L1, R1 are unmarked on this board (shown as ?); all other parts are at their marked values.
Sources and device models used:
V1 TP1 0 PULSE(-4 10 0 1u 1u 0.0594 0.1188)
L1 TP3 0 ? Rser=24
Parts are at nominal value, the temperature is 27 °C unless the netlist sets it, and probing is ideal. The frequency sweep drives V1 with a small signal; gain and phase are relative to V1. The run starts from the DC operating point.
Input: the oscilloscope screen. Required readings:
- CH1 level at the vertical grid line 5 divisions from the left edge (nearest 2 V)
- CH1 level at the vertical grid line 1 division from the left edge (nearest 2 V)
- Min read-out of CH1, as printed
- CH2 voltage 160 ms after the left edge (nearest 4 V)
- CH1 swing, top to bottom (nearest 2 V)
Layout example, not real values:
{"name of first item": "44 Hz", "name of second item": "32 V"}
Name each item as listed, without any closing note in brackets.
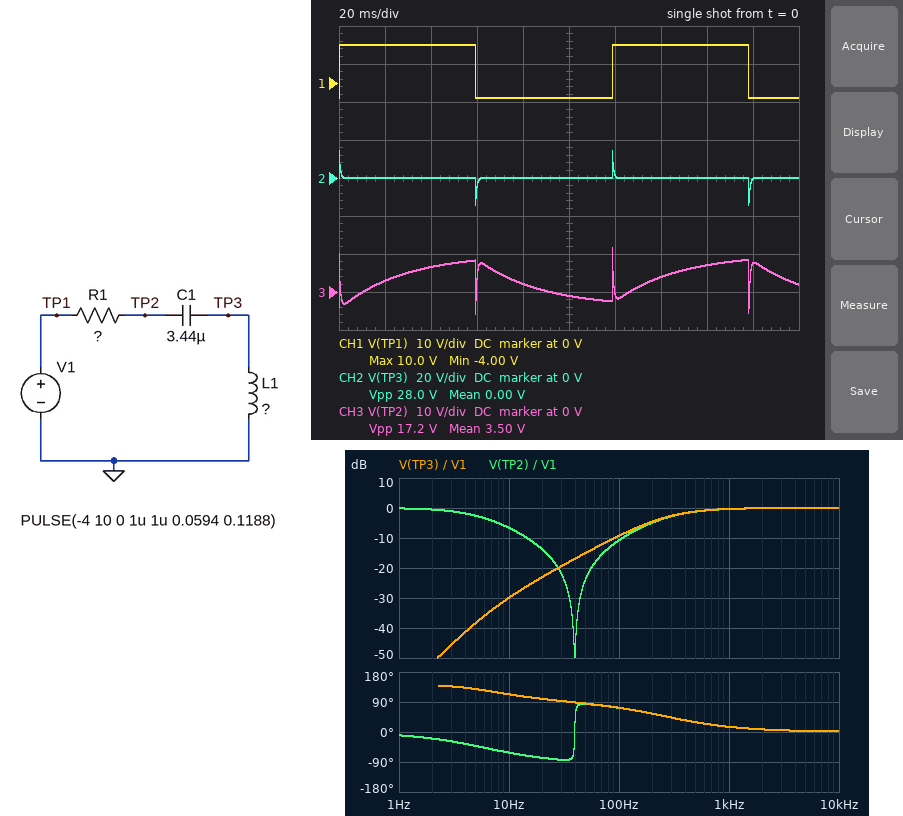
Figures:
{"CH1 level at the vertical grid line 5 divisions from the left edge": "-4 V", "CH1 level at the vertical grid line 1 division from the left edge": "10 V", "Min read-out of CH1, as printed": "-4.00 V", "CH2 voltage 160 ms after the left edge": "0 V", "CH1 swing, top to bottom": "14 V"}
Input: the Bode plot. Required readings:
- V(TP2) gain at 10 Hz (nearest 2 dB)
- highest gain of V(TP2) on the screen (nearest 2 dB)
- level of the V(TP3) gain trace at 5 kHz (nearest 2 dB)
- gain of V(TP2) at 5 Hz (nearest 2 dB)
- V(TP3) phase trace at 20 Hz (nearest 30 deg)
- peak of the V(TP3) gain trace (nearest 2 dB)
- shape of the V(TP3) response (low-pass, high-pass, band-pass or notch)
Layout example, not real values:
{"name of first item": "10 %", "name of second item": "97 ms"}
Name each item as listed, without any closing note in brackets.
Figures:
{"V(TP2) gain at 10 Hz": "-6 dB", "highest gain of V(TP2) on the screen": "0 dB", "level of the V(TP3) gain trace at 5 kHz": "0 dB", "gain of V(TP2) at 5 Hz": "-2 dB", "V(TP3) phase trace at 20 Hz": "90 deg", "peak of the V(TP3) gain trace": "0 dB", "shape of the V(TP3) response": "high-pass"}
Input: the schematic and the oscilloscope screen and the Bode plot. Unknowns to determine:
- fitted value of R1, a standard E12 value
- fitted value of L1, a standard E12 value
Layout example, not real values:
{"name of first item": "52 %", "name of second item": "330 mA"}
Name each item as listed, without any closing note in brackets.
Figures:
{"fitted value of R1, a standard E12 value": "8.2 kΩ", "fitted value of L1, a standard E12 value": "4.7 H"}
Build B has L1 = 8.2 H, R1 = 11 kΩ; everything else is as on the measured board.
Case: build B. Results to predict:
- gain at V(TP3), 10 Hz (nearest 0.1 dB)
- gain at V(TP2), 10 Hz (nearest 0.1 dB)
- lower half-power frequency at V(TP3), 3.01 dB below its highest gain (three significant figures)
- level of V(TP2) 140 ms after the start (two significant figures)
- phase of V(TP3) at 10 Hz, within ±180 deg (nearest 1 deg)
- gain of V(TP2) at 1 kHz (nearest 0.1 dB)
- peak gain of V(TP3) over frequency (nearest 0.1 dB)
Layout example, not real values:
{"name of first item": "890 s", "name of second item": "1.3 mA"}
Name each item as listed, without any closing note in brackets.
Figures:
{"gain at V(TP3), 10 Hz": "-27.2 dB", "gain at V(TP2), 10 Hz": "-9.1 dB", "lower half-power frequency at V(TP3), 3.01 dB below its highest gain": "210 Hz", "level of V(TP2) 140 ms after the start": "3.1 V", "phase of V(TP3) at 10 Hz, within ±180 deg": "108 deg", "gain of V(TP2) at 1 kHz": "-0.2 dB", "peak gain of V(TP3) over frequency": "0 dB"}
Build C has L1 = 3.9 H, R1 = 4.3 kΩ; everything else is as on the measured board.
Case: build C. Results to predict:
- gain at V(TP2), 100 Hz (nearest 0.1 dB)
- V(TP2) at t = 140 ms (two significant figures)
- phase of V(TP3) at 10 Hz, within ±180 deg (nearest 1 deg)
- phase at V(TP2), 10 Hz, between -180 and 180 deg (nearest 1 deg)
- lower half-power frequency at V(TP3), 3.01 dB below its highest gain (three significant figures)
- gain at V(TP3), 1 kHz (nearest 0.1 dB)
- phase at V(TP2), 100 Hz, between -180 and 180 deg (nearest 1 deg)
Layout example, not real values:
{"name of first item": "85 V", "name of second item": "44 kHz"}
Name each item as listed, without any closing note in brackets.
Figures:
{"gain at V(TP2), 100 Hz": "-7.6 dB", "V(TP2) at t = 140 ms": "6.6 V", "phase of V(TP3) at 10 Hz, within ±180 deg": "130 deg", "phase at V(TP2), 10 Hz, between -180 and 180 deg": "-44 deg", "lower half-power frequency at V(TP3), 3.01 dB below its highest gain": "166 Hz", "gain at V(TP3), 1 kHz": "-0.1 dB", "phase at V(TP2), 100 Hz, between -180 and 180 deg": "65 deg"}
